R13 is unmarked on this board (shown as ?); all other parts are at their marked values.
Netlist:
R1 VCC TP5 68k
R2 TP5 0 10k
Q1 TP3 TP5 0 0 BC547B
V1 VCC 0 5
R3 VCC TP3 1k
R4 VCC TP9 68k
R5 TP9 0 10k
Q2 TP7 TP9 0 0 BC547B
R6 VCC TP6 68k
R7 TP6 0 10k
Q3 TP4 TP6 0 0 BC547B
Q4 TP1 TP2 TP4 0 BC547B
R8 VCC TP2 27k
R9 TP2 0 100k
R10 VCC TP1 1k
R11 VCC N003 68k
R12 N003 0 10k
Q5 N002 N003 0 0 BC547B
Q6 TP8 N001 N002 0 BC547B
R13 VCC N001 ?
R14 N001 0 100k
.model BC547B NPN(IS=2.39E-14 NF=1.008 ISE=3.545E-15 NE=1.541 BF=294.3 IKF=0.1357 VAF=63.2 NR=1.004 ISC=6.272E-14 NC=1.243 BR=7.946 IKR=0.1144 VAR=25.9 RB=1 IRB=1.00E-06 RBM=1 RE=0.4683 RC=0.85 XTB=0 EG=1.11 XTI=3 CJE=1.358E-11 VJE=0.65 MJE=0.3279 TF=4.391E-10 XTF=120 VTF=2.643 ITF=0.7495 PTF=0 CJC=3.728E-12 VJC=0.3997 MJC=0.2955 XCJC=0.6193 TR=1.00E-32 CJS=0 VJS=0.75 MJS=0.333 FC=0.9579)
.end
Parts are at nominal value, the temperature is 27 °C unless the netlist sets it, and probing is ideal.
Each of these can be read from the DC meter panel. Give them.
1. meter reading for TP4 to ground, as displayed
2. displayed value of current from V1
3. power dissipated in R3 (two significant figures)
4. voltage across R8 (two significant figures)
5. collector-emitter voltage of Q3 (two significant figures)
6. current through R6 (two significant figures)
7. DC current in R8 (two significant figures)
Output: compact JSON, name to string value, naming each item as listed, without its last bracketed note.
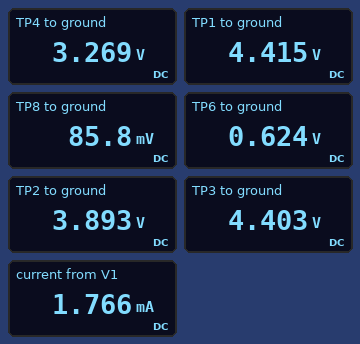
{"meter reading for TP4 to ground, as displayed": "3.269 V", "displayed value of current from V1": "1.766 mA", "power dissipated in R3": "360 µW", "voltage across R8": "1.1 V", "collector-emitter voltage of Q3": "3.3 V", "current through R6": "64 µA", "DC current in R8": "41 µA"}
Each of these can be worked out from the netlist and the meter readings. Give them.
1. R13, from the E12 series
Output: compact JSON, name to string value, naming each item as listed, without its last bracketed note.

{"R13, from the E12 series": "15 kΩ"}
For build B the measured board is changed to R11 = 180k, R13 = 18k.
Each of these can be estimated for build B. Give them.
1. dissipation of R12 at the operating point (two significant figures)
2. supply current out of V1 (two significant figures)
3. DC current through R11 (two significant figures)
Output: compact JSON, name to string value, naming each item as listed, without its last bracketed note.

{"dissipation of R12 at the operating point": "6.9 µW", "supply current out of V1": "1.5 mA", "DC current through R11": "26 µA"}
